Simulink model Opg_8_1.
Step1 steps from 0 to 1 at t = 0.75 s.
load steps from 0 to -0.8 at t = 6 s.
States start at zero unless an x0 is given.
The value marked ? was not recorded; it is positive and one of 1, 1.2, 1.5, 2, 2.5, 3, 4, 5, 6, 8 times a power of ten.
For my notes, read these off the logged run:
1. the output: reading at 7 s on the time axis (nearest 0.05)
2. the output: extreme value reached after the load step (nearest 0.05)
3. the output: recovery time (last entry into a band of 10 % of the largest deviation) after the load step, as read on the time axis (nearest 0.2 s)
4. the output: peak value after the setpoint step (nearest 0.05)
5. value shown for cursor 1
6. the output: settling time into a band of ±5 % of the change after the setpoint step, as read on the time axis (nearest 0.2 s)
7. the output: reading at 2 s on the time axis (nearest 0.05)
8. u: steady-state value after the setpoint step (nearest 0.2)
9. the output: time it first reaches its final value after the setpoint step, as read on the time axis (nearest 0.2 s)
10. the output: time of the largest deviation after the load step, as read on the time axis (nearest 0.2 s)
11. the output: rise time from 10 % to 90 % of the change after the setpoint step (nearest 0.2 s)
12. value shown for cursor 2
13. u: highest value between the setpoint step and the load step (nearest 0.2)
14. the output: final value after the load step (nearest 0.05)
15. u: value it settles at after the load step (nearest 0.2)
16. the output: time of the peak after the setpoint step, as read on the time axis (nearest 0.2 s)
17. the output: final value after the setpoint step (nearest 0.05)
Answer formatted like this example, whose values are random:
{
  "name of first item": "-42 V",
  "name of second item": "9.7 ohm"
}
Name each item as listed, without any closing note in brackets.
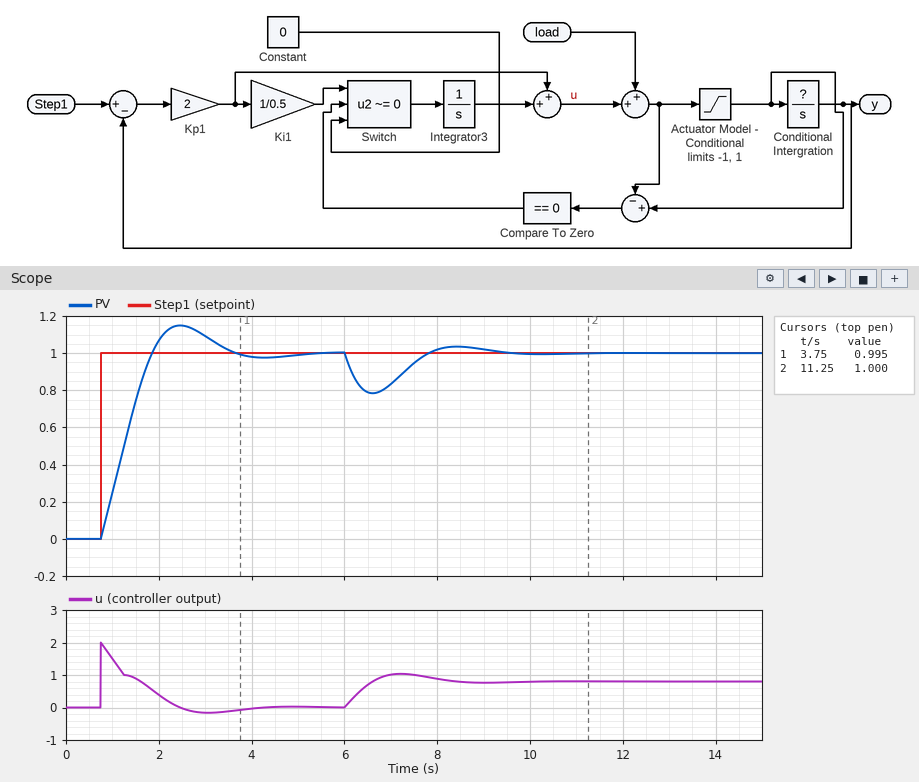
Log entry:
{
  "the output: reading at 7 s on the time axis": "0.85",
  "the output: extreme value reached after the load step": "0.80",
  "the output: recovery time (last entry into a band of 10 % of the largest deviation) after the load step, as read on the time axis": "9.0 s",
  "the output: peak value after the setpoint step": "1.15",
  "value shown for cursor 1": "0.995",
  "the output: settling time into a band of ±5 % of the change after the setpoint step, as read on the time axis": "3.2 s",
  "the output: reading at 2 s on the time axis": "1.05",
  "u: steady-state value after the setpoint step": "0.0",
  "the output: time it first reaches its final value after the setpoint step, as read on the time axis": "1.8 s",
  "the output: time of the largest deviation after the load step, as read on the time axis": "6.6 s",
  "the output: rise time from 10 % to 90 % of the change after the setpoint step": "0.8 s",
  "value shown for cursor 2": "1.000",
  "u: highest value between the setpoint step and the load step": "2.0",
  "the output: final value after the load step": "1.00",
  "u: value it settles at after the load step": "0.8",
  "the output: time of the peak after the setpoint step, as read on the time axis": "2.4 s",
  "the output: final value after the setpoint step": "1.00"
}
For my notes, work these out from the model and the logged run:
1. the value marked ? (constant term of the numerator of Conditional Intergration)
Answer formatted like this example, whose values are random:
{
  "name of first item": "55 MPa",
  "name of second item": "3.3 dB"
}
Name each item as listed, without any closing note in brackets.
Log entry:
{
  "the value marked ?": "1"
}
